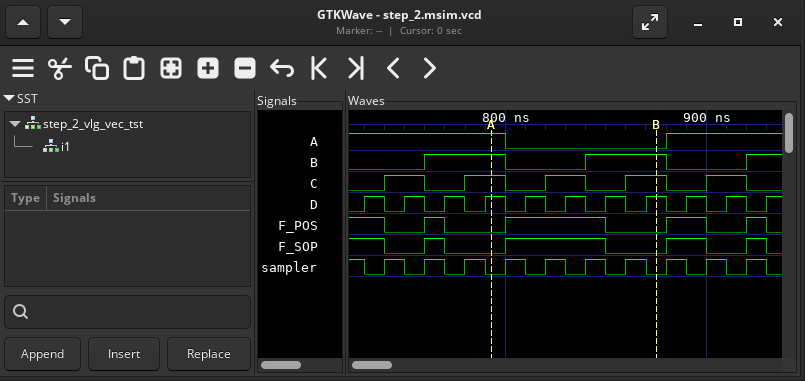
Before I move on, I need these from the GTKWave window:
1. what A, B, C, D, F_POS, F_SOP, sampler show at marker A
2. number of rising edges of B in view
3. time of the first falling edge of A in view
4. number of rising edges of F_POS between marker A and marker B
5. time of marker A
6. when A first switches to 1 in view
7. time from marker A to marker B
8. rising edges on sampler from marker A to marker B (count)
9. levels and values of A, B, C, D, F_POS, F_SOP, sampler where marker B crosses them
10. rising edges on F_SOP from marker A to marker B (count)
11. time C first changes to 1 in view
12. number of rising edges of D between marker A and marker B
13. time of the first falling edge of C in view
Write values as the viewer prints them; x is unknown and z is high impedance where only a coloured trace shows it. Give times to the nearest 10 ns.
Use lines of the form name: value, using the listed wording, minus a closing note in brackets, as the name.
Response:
what A, B, C, D, F_POS, F_SOP, sampler show at marker A: A=1, B=1, C=1, D=1, F_POS=0, F_SOP=0, sampler=0
number of rising edges of B in view: 3
time of the first falling edge of A in view: 800 ns
number of rising edges of F_POS between marker A and marker B: 1
time of marker A: 790 ns
when A first switches to 1 in view: 880 ns
time from marker A to marker B: 80 ns
rising edges on sampler from marker A to marker B: 4
levels and values of A, B, C, D, F_POS, F_SOP, sampler where marker B crosses them: A=0, B=1, C=1, D=1, F_POS=0, F_SOP=0, sampler=0
rising edges on F_SOP from marker A to marker B: 1
time C first changes to 1 in view: 740 ns
number of rising edges of D between marker A and marker B: 4
time of the first falling edge of C in view: 760 ns
